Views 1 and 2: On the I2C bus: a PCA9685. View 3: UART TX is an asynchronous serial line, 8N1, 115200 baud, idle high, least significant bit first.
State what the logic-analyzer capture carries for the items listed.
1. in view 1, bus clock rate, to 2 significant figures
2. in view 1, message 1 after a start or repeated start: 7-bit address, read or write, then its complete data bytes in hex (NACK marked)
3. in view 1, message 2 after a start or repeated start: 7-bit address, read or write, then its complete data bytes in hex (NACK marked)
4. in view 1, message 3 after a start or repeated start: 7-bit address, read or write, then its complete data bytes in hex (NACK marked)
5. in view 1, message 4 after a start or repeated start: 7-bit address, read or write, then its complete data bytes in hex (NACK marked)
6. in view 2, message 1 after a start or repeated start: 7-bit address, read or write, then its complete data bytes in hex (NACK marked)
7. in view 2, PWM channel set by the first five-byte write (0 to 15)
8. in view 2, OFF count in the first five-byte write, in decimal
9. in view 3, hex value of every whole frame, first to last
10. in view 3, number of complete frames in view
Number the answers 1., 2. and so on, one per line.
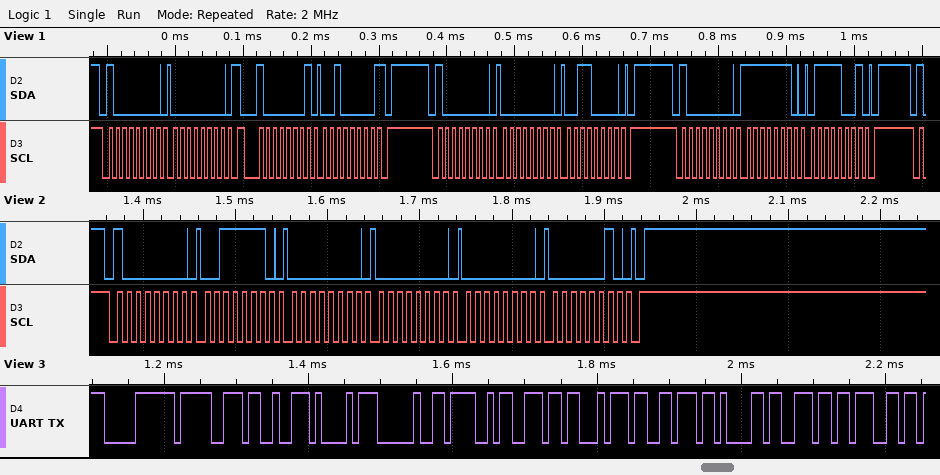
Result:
1. 100 kHz
2. 0x40 write: 00
3. 0x40 read: 20 NACK
4. 0x40 write: 00 30
5. 0x40 write: FE 79
6. 0x40 write: 3E 00 00 00 02
7. 14
8. 512
9. F0 9F 93 A1 20 4F 6E 74 76 61 6E 67
10. 12
